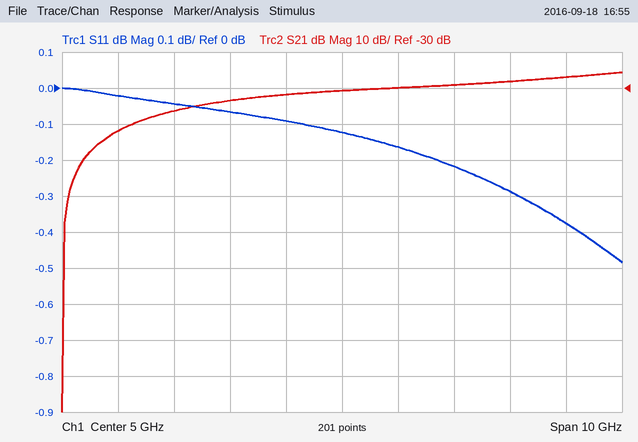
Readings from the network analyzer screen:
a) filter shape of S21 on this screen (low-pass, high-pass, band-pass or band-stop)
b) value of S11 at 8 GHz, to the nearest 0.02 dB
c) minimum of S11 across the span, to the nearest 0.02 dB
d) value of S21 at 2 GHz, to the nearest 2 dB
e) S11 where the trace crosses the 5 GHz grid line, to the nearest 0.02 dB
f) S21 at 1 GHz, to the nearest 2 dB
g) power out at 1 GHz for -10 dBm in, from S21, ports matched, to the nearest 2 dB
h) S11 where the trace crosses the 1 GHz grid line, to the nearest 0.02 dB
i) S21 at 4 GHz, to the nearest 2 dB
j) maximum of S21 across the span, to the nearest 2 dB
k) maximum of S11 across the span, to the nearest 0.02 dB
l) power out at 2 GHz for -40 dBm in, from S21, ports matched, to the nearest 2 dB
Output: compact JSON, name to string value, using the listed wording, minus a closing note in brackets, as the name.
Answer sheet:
{"filter shape of S21 on this screen": "high-pass", "value of S11 at 8 GHz, to the nearest 0.02 dB": "-0.28 dB", "minimum of S11 across the span, to the nearest 0.02 dB": "-0.48 dB", "value of S21 at 2 GHz, to the nearest 2 dB": "-36 dB", "S11 where the trace crosses the 5 GHz grid line, to the nearest 0.02 dB": "-0.12 dB", "S21 at 1 GHz, to the nearest 2 dB": "-42 dB", "power out at 1 GHz for -10 dBm in, from S21, ports matched, to the nearest 2 dB": "-52 dBm", "S11 where the trace crosses the 1 GHz grid line, to the nearest 0.02 dB": "-0.02 dB", "S21 at 4 GHz, to the nearest 2 dB": "-32 dB", "maximum of S21 across the span, to the nearest 2 dB": "-26 dB", "maximum of S11 across the span, to the nearest 0.02 dB": "0.00 dB", "power out at 2 GHz for -40 dBm in, from S21, ports matched, to the nearest 2 dB": "-76 dBm"}
